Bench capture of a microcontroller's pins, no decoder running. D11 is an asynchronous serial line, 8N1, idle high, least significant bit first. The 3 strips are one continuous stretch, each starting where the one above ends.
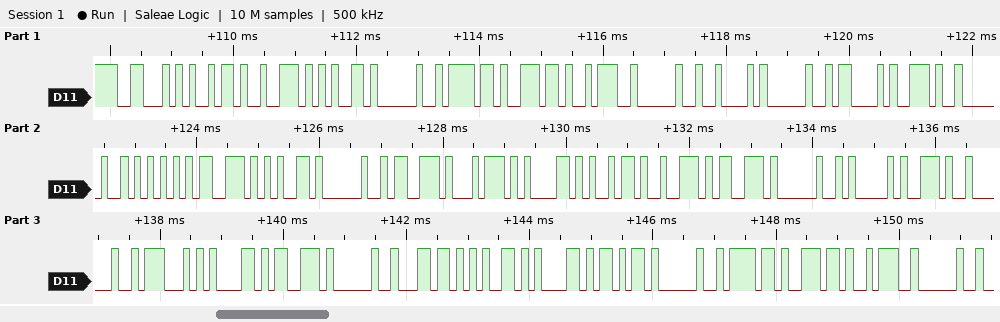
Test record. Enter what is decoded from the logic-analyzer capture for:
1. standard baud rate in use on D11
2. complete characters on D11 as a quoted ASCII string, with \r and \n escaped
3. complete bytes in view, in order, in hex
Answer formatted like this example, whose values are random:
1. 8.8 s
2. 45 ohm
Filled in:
1. 9600 baud
2. "Fire on: B C. Use stairs A. Gas leak on: "
3. 46 69 72 65 20 6F 6E 3A 20 42 20 43 2E 20 55 73 65 20 73 74 61 69 72 73 20 41 2E 20 47 61 73 20 6C 65 61 6B 20 6F 6E 3A 20
